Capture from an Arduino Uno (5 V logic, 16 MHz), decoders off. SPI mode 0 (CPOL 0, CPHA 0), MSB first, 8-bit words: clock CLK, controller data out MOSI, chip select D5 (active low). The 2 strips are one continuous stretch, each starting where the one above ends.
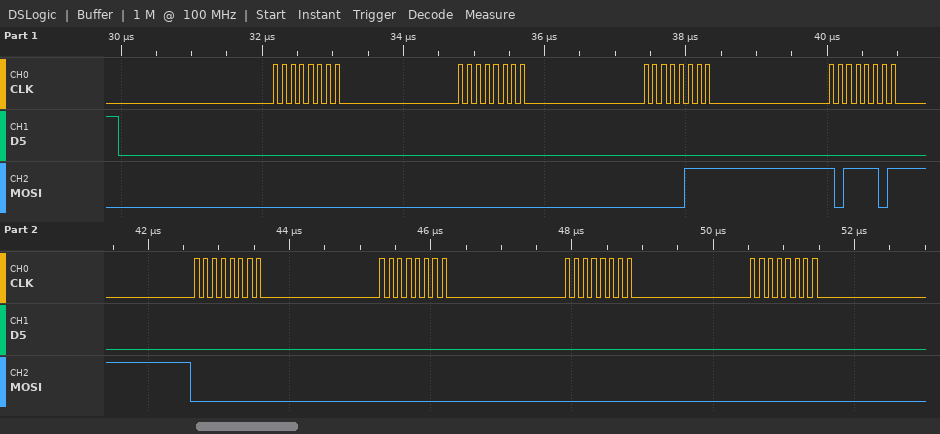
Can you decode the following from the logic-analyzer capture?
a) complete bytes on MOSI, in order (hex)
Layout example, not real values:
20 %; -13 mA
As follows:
0x00 0x00 0x07 0xBD 0x00 0x00 0x00 0x00
